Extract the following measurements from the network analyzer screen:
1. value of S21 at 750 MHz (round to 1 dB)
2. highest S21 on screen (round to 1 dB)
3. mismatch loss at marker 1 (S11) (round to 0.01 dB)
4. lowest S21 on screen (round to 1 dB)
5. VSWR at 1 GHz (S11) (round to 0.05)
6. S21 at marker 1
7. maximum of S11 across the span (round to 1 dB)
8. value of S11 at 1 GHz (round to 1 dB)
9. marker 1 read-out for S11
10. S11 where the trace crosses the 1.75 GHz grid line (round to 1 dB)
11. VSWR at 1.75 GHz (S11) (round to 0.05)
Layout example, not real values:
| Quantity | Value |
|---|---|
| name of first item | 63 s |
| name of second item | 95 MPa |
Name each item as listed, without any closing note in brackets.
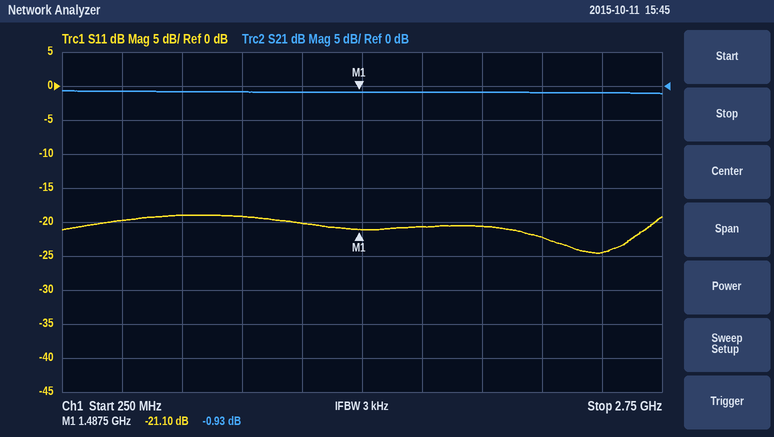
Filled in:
| Quantity | Value |
|---|---|
| value of S21 at 750 MHz | -1 dB |
| highest S21 on screen | -1 dB |
| mismatch loss at marker 1 (S11) | 0.03 dB |
| lowest S21 on screen | -1 dB |
| VSWR at 1 GHz (S11) | 1.25 |
| S21 at marker 1 | -0.93 dB |
| maximum of S11 across the span | -19 dB |
| value of S11 at 1 GHz | -19 dB |
| marker 1 read-out for S11 | -21.10 dB |
| S11 where the trace crosses the 1.75 GHz grid line | -21 dB |
| VSWR at 1.75 GHz (S11) | 1.20 |
